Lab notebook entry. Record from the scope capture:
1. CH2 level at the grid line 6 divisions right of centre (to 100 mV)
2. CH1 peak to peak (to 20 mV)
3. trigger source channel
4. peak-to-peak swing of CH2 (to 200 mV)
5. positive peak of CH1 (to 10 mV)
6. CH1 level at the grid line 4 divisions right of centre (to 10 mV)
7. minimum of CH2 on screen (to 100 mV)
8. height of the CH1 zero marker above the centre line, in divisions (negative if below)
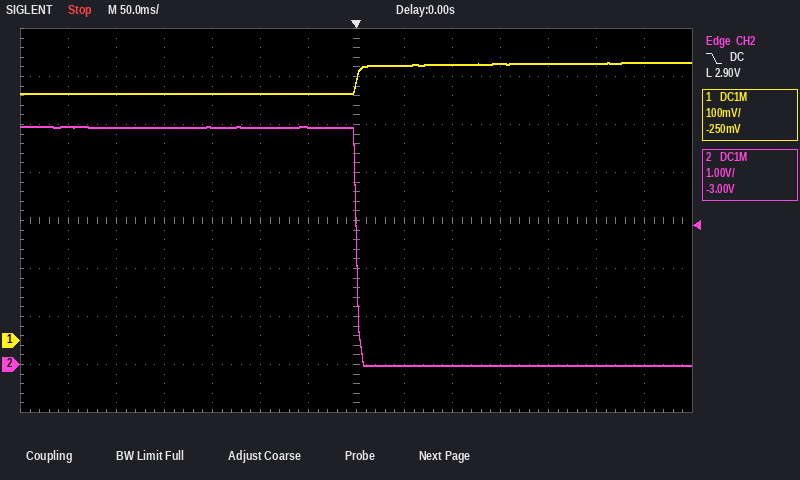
0.0 V
60 mV
CH2
5.0 V
580 mV
580 mV
0.0 V
-2.5 div
